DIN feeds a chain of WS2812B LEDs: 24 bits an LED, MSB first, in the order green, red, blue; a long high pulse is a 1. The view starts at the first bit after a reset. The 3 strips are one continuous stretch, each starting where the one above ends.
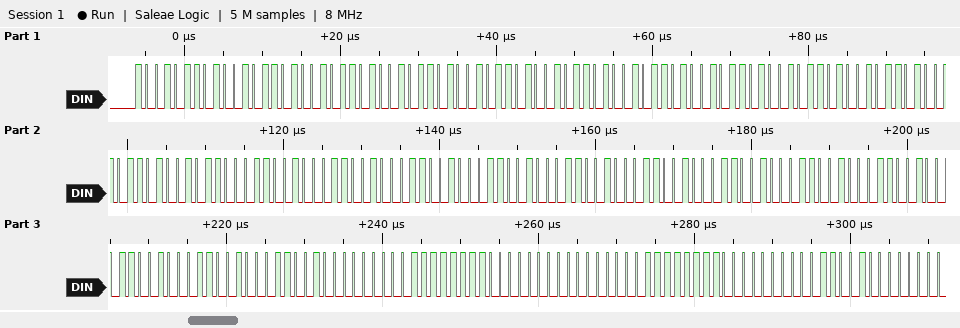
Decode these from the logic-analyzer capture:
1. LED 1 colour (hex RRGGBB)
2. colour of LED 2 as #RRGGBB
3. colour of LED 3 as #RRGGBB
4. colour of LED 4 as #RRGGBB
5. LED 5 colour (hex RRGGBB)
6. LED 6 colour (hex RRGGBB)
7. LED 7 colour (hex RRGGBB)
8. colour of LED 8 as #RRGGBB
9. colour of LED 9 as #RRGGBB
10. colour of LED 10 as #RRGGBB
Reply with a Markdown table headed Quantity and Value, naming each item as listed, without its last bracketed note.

| Quantity | Value |
|---|---|
| LED 1 colour | #969696 |
| colour of LED 2 as #RRGGBB | #969696 |
| colour of LED 3 as #RRGGBB | #969696 |
| colour of LED 4 as #RRGGBB | #969696 |
| LED 5 colour | #323232 |
| LED 6 colour | #323232 |
| LED 7 colour | #323232 |
| colour of LED 8 as #RRGGBB | #323232 |
| colour of LED 9 as #RRGGBB | #FF0000 |
| colour of LED 10 as #RRGGBB | #FF0000 |
